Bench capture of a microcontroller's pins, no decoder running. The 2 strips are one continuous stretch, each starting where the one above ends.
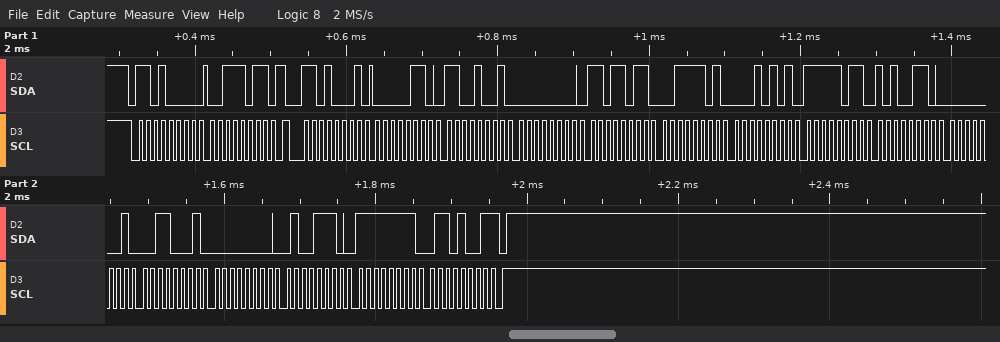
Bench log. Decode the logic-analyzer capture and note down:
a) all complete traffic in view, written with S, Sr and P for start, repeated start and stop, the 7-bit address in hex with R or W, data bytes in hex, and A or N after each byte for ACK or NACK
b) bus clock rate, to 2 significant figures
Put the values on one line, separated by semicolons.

S 68W A 3B A Sr 68R A 06 A C9 A 00 A DB A 3D A 15 A FB A A6 A 01 A 31 A 00 A 4E A FF A 69 N P; 100 kHz
